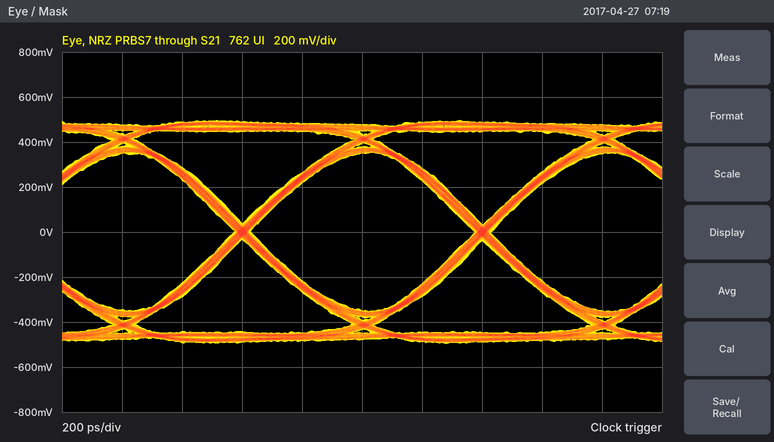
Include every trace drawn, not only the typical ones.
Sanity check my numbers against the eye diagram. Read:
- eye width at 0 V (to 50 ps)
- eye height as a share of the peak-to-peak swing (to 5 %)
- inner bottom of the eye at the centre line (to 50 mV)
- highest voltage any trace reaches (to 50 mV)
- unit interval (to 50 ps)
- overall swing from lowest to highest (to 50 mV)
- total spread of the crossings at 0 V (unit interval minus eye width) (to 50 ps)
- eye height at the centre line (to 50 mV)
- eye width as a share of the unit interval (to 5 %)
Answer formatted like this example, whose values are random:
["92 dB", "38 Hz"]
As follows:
["750 ps", "70 %", "-350 mV", "500 mV", "800 ps", "1.00 V", "50 ps", "700 mV", "95 %"]
